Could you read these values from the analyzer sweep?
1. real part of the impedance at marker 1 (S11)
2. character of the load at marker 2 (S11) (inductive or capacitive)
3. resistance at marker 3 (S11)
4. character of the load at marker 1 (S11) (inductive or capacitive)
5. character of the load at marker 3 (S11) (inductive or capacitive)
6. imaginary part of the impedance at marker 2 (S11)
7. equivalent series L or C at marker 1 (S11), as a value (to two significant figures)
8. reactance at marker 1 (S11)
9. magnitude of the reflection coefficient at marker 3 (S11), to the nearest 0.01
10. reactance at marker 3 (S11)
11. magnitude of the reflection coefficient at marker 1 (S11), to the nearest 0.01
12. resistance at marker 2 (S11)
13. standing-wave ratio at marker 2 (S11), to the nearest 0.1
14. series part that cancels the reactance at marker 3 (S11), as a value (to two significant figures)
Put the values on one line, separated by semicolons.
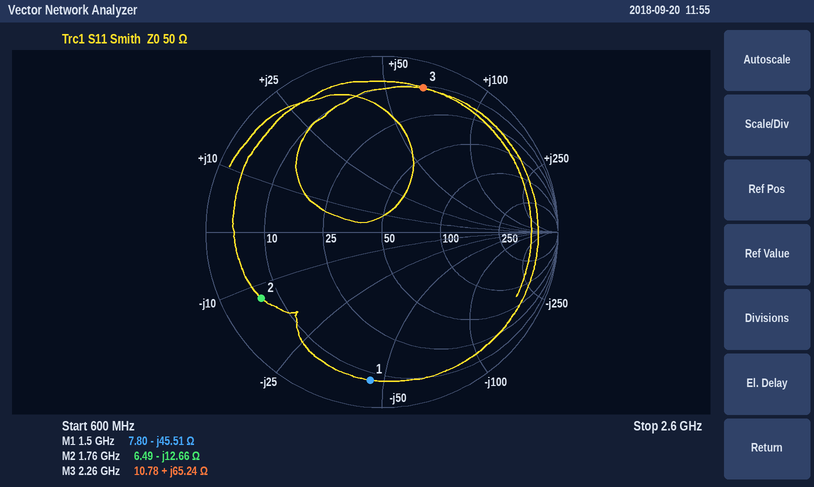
7.80 Ω; capacitive; 10.78 Ω; capacitive; inductive; -12.66 Ω; 2.3 pF; -45.51 Ω; 0.85; +65.24 Ω; 0.84; 6.49 Ω; 8.2; 1.1 pF
